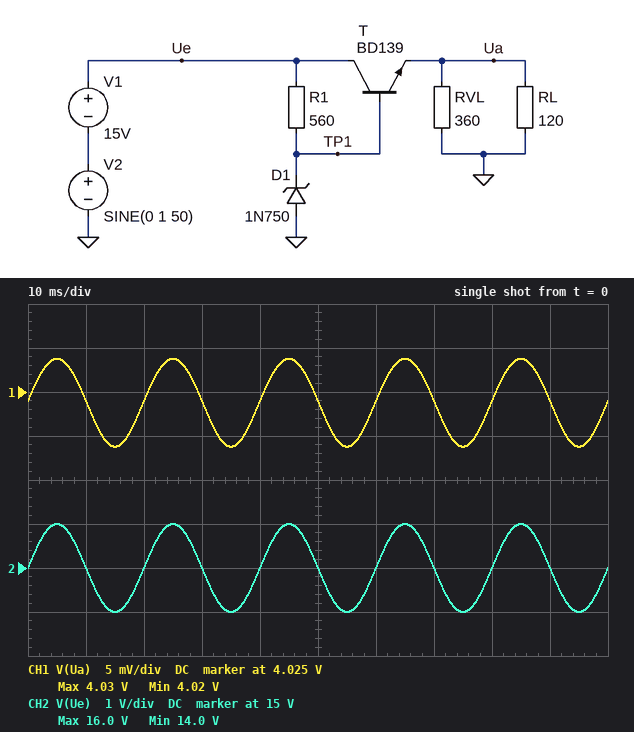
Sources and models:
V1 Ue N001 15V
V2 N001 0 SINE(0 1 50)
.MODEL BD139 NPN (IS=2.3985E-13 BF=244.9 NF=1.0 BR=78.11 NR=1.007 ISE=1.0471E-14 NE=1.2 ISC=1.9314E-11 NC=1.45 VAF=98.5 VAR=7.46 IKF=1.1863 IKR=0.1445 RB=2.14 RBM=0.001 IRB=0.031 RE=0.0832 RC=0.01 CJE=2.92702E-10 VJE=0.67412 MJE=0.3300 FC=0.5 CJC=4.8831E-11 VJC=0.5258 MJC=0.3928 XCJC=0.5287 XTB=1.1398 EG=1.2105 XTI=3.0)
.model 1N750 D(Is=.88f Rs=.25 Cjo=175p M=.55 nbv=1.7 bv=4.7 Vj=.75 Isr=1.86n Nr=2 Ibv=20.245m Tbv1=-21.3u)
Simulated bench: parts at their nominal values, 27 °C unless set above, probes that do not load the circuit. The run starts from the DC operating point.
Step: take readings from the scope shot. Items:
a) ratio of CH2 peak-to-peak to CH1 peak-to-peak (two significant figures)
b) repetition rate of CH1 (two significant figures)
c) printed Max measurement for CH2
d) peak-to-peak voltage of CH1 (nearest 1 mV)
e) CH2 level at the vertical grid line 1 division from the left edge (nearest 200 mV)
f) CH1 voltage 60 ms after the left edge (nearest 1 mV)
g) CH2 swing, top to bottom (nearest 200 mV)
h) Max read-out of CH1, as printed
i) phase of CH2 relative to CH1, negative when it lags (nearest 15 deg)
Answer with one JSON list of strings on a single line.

["200", "50 Hz", "16.0 V", "10 mV", "15.0 V", "4.024 V", "2.0 V", "4.03 V", "0 deg"]
